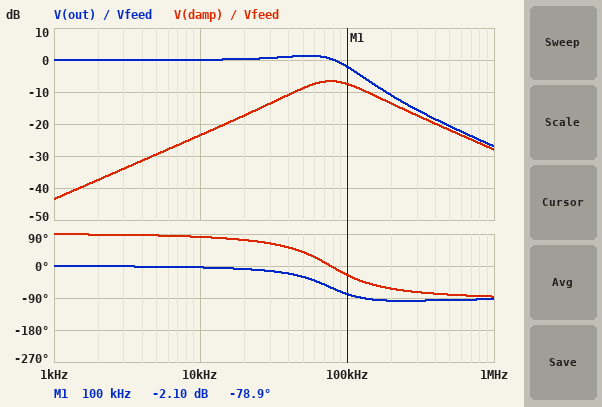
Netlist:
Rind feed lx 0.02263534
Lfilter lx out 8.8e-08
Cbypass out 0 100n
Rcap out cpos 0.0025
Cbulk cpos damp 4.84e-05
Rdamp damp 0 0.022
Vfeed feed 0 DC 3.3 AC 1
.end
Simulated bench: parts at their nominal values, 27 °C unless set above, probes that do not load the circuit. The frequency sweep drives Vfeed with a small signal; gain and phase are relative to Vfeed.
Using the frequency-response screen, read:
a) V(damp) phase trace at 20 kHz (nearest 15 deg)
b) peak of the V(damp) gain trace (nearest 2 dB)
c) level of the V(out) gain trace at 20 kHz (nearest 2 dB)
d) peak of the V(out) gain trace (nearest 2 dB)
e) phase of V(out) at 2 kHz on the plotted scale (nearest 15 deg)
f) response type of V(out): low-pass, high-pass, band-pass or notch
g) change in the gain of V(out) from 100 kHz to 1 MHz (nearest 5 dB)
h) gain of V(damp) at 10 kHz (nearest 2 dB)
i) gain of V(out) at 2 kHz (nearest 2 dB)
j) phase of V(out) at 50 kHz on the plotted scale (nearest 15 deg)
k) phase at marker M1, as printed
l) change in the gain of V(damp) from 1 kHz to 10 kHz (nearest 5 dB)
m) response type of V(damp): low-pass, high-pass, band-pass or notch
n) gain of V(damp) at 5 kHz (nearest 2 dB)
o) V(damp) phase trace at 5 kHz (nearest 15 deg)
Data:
75 deg
-6 dB
0 dB
2 dB
0 deg
low-pass
-25 dB
-24 dB
0 dB
-30 deg
-78.9 deg
20 dB
band-pass
-30 dB
90 deg
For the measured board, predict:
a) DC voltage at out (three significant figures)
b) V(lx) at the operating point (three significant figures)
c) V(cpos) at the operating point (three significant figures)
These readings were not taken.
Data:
3.30 V
3.30 V
3.30 V
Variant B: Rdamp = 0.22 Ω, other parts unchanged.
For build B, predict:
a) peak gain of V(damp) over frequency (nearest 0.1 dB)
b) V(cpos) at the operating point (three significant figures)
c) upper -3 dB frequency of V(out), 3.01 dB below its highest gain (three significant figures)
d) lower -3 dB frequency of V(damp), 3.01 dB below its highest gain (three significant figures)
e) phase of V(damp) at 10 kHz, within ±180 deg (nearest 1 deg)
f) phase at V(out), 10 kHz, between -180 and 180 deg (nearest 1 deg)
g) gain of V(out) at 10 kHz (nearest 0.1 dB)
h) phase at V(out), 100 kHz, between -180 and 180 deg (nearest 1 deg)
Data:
-0.9 dB
3.30 V
395 kHz
13.1 kHz
53 deg
-3 deg
-0.2 dB
-14 deg
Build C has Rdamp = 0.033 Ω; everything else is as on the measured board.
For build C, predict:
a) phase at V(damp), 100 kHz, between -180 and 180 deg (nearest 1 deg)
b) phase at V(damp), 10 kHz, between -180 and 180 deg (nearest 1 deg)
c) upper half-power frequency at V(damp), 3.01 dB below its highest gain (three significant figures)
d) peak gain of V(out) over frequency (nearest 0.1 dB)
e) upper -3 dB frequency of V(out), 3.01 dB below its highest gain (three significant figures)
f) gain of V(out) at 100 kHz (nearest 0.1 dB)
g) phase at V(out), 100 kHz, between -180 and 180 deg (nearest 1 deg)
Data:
-21 deg
80 deg
146 kHz
0.6 dB
102 kHz
-2.2 dB
-64 deg
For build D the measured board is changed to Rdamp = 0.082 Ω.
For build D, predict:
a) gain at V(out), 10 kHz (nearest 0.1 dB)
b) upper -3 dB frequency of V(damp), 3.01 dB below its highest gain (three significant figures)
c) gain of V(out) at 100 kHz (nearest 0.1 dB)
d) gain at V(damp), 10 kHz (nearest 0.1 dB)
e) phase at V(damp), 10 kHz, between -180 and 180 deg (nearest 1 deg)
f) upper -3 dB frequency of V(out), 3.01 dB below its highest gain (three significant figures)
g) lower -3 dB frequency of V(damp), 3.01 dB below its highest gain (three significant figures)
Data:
0 dB
222 kHz
-1.6 dB
-12.4 dB
72 deg
151 kHz
27.0 kHz
